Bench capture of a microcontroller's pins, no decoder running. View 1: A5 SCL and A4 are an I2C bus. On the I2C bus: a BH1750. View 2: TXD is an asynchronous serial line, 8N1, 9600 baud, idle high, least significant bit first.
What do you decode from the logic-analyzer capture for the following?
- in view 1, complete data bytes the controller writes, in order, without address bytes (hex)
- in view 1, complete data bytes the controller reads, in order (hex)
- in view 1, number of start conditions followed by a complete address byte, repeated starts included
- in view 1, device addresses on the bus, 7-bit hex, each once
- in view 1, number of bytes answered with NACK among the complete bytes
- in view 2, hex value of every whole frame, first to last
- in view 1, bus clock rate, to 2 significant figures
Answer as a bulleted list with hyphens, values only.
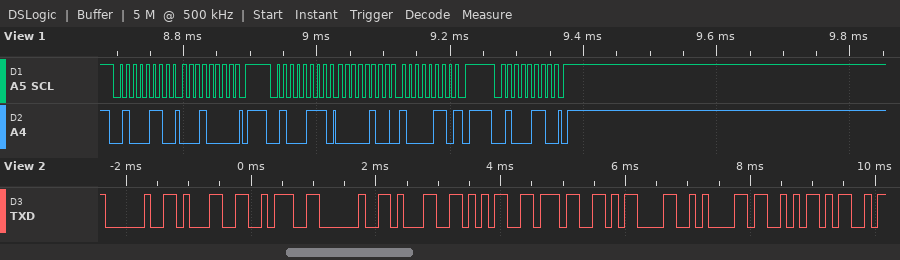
- 10
- 04 86
- 3
- 0x23
- 1
- 0x20 0x31 0x3A 0x20 0x31 0x35 0x37 0x0D 0x0A 0x53 0x4D
- 100 kHz
